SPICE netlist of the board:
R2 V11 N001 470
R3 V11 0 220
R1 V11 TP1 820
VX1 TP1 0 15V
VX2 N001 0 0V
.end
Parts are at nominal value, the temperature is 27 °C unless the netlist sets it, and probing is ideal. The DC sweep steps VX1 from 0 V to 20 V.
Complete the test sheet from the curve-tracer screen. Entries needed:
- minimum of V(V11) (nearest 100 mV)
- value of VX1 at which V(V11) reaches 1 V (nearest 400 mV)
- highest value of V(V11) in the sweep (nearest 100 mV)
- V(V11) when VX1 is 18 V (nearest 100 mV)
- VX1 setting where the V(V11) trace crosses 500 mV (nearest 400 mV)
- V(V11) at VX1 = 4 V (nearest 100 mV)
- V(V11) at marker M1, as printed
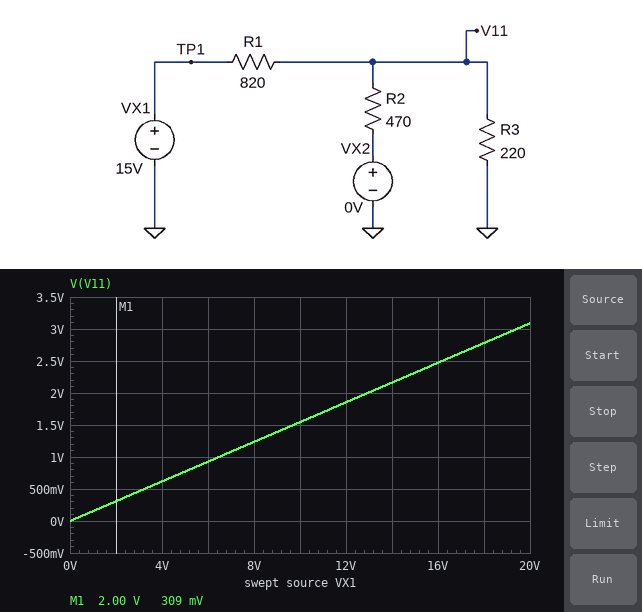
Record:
0 V
6.4 V
3.1 V
2.8 V
3.2 V
600 mV
309 mV
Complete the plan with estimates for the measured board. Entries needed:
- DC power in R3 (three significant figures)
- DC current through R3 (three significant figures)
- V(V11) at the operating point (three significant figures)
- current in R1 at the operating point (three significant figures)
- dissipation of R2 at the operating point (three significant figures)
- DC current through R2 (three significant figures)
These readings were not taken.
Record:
24.4 mW
10.5 mA
2.32 V
15.5 mA
11.4 mW
4.93 mA
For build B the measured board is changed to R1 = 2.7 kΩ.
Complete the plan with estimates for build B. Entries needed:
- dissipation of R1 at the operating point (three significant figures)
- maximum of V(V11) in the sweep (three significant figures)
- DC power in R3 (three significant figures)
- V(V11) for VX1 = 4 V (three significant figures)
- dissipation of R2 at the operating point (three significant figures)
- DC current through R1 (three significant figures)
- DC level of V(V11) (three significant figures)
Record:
74.8 mW
1.05 V
2.83 mW
210 mV
1.32 mW
5.26 mA
789 mV
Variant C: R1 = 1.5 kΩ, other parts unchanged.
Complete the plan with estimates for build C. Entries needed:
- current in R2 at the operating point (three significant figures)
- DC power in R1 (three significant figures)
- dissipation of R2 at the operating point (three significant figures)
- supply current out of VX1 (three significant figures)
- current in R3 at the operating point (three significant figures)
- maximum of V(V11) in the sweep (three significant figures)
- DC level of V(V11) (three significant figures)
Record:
2.90 mA
124 mW
3.95 mW
9.09 mA
6.19 mA
1.82 V
1.36 V
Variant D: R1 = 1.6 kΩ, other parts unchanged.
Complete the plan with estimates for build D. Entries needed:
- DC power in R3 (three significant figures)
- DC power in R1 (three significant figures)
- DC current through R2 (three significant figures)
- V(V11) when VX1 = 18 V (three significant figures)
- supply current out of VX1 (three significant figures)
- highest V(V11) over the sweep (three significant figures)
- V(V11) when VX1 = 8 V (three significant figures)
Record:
7.50 mW
118 mW
2.73 mA
1.54 V
8.57 mA
1.71 V
685 mV
